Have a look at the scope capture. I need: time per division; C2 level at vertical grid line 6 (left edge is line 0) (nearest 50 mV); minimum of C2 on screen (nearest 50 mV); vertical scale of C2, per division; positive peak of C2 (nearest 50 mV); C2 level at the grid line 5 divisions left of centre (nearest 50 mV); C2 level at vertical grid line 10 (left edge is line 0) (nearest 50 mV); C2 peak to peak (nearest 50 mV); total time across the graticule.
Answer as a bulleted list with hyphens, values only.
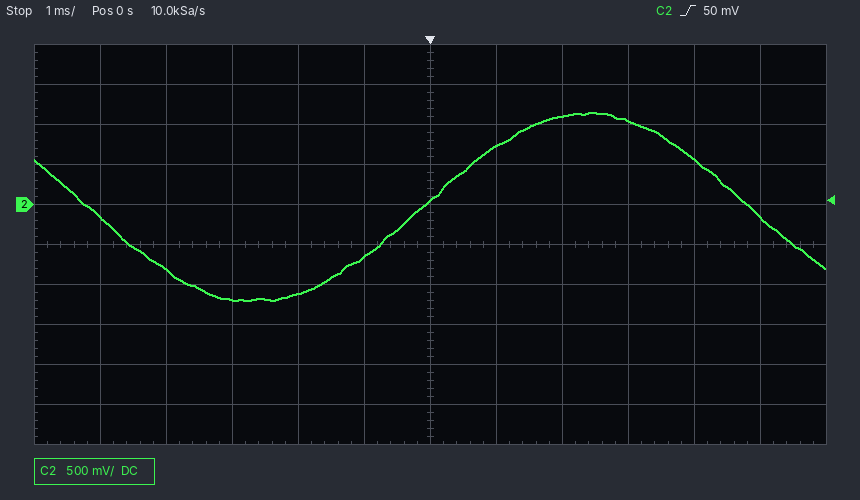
- 1 ms
- 50 mV
- -1.20 V
- 500 mV
- 1.15 V
- -150 mV
- 550 mV
- 2.35 V
- 12 ms
